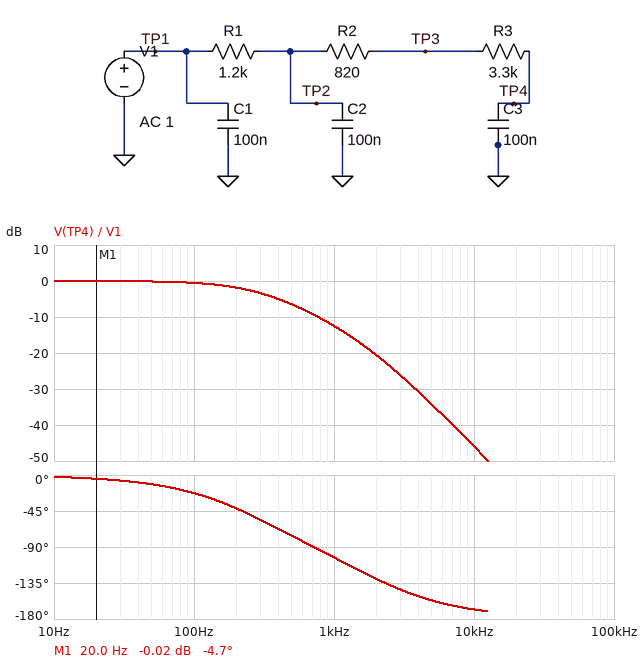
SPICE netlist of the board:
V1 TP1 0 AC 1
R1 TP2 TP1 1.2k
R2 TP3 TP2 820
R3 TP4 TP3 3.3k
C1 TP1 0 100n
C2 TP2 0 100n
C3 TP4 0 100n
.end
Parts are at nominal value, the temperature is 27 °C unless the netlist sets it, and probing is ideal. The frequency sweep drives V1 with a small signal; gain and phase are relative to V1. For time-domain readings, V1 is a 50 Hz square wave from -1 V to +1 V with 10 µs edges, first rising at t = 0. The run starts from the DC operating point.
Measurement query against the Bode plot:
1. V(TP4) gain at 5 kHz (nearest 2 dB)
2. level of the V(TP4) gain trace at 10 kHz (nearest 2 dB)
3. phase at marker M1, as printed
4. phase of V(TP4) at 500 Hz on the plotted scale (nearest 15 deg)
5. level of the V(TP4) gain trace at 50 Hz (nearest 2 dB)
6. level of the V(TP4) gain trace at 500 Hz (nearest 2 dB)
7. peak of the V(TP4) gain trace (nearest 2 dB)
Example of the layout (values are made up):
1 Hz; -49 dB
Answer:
-34 dB; -46 dB; -4.7 deg; -75 deg; 0 dB; -6 dB; 0 dB
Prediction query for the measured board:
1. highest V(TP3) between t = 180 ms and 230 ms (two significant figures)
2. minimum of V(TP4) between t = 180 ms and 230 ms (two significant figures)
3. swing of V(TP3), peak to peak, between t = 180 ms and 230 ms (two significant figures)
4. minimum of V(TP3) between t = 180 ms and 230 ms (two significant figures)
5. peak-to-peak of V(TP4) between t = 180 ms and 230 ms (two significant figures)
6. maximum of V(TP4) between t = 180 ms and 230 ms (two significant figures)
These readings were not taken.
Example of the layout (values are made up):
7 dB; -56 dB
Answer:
1.0 V; -1.0 V; 2.0 V; -1.0 V; 2.0 V; 1.0 V
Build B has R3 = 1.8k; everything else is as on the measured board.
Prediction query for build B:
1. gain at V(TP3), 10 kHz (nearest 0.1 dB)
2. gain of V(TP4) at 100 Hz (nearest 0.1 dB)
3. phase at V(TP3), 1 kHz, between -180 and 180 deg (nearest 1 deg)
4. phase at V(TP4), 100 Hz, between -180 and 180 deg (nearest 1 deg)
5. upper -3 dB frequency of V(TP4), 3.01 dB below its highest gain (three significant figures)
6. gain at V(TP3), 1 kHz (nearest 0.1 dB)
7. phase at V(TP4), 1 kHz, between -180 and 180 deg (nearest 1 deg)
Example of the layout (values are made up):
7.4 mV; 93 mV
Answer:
-21.0 dB; -0.3 dB; -46 deg; -18 deg; 361 Hz; -6.4 dB; -94 deg
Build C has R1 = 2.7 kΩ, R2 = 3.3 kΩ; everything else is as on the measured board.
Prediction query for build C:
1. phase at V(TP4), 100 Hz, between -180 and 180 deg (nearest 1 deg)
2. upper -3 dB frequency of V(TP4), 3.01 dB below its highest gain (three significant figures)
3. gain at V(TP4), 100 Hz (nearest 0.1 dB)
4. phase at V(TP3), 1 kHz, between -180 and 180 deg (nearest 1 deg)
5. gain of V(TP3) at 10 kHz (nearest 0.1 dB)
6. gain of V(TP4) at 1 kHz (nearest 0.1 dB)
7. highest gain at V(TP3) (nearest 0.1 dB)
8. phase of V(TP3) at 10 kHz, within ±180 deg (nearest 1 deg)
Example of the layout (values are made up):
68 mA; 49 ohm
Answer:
-39 deg; 151 Hz; -1.6 dB; -64 deg; -30.6 dB; -19.7 dB; 0 dB; -87 deg
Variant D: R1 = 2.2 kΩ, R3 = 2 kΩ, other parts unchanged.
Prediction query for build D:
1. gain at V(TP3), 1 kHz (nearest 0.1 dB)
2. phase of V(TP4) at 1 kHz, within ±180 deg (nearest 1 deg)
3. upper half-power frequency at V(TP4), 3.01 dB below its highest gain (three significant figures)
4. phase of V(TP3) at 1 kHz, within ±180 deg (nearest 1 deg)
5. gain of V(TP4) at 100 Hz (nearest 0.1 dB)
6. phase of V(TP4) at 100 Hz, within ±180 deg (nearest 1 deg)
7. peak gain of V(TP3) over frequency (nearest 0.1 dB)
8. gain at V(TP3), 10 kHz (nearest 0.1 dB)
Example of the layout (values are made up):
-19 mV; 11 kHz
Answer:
-9.4 dB; -108 deg; 250 Hz; -56 deg; -0.6 dB; -25 deg; 0 dB; -25.9 dB
